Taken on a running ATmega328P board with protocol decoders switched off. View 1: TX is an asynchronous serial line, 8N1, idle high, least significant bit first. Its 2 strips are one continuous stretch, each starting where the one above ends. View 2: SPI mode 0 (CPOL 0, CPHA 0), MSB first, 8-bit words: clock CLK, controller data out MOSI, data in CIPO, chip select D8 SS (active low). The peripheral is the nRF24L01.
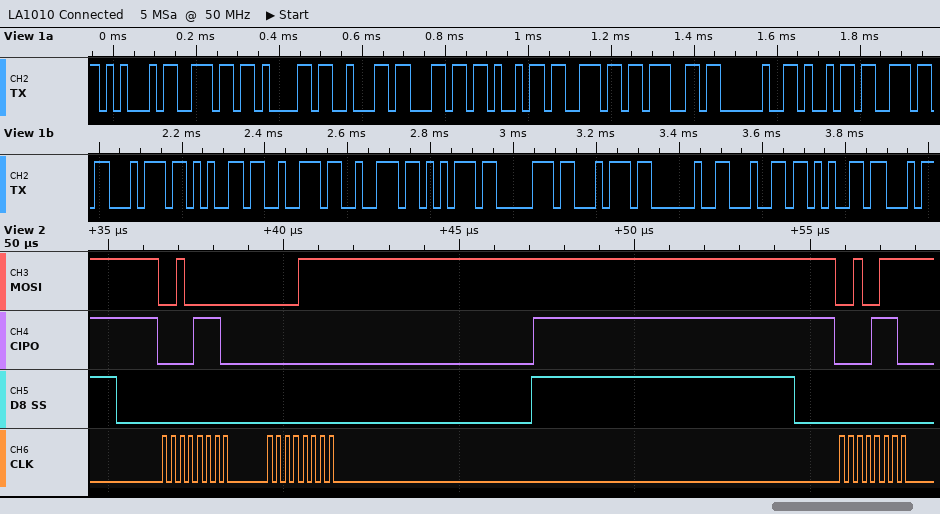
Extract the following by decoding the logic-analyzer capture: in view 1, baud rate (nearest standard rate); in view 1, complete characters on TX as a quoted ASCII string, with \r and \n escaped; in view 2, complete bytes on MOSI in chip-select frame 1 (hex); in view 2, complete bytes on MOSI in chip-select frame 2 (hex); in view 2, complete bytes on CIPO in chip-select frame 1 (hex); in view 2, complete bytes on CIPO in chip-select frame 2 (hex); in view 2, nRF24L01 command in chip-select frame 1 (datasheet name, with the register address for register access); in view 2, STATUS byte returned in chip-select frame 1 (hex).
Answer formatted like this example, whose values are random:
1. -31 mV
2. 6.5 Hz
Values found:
1. 57600 baud
2. "Enabling interrupt de"
3. 0x20 0x0F
4. 0x27
5. 0x0E 0x00
6. 0x0E
7. W_REGISTER 0x00
8. 0x0E
